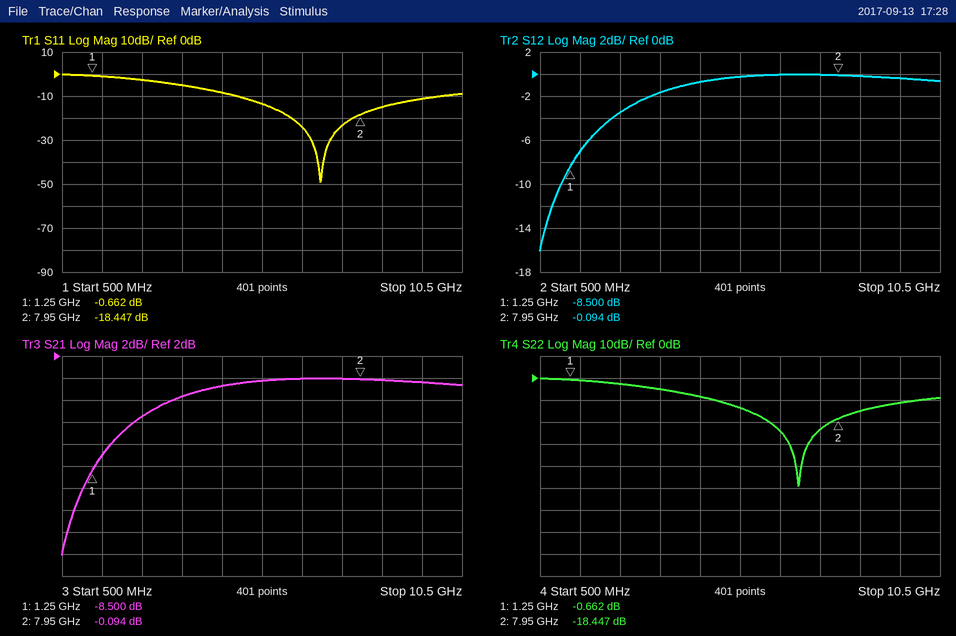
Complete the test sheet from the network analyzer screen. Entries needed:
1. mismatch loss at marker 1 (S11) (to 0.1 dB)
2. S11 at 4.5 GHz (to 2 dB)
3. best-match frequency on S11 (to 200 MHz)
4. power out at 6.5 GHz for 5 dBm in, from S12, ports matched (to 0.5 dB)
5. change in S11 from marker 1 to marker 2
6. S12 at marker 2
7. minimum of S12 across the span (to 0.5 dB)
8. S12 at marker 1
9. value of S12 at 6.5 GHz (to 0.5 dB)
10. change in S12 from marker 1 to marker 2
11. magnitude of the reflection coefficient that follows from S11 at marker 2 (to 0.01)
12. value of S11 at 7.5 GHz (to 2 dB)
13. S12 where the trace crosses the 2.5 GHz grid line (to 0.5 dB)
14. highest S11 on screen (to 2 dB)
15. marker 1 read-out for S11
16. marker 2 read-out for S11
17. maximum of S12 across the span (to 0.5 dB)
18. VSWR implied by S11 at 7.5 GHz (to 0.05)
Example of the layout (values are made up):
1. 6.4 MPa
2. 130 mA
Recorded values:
1. 8.5 dB
2. -8 dB
3. 7.0 GHz
4. 5.0 dBm
5. -17.785 dB
6. -0.094 dB
7. -16.0 dB
8. -8.500 dB
9. 0.0 dB
10. 8.406 dB
11. 0.12
12. -24 dB
13. -3.5 dB
14. 0 dB
15. -0.662 dB
16. -18.447 dB
17. 0.0 dB
18. 1.15
